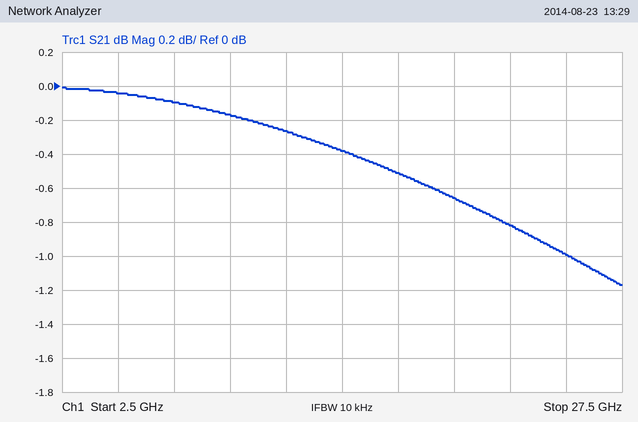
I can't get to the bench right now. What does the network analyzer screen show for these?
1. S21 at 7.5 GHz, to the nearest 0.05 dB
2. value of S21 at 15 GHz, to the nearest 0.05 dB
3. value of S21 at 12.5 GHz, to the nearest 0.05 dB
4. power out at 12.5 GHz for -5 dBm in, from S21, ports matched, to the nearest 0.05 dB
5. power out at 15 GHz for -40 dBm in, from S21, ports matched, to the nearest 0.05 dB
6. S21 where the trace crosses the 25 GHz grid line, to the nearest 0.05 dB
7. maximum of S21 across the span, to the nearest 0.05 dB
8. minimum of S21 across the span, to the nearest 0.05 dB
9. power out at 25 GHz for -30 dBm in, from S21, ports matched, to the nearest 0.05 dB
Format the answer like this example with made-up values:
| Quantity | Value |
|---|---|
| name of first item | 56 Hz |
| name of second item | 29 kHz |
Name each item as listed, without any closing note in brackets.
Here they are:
| Quantity | Value |
|---|---|
| S21 at 7.5 GHz, to the nearest 0.05 dB | -0.10 dB |
| value of S21 at 15 GHz, to the nearest 0.05 dB | -0.40 dB |
| value of S21 at 12.5 GHz, to the nearest 0.05 dB | -0.25 dB |
| power out at 12.5 GHz for -5 dBm in, from S21, ports matched, to the nearest 0.05 dB | -5.25 dBm |
| power out at 15 GHz for -40 dBm in, from S21, ports matched, to the nearest 0.05 dB | -40.40 dBm |
| S21 where the trace crosses the 25 GHz grid line, to the nearest 0.05 dB | -1.00 dB |
| maximum of S21 across the span, to the nearest 0.05 dB | 0.00 dB |
| minimum of S21 across the span, to the nearest 0.05 dB | -1.15 dB |
| power out at 25 GHz for -30 dBm in, from S21, ports matched, to the nearest 0.05 dB | -31.00 dBm |
